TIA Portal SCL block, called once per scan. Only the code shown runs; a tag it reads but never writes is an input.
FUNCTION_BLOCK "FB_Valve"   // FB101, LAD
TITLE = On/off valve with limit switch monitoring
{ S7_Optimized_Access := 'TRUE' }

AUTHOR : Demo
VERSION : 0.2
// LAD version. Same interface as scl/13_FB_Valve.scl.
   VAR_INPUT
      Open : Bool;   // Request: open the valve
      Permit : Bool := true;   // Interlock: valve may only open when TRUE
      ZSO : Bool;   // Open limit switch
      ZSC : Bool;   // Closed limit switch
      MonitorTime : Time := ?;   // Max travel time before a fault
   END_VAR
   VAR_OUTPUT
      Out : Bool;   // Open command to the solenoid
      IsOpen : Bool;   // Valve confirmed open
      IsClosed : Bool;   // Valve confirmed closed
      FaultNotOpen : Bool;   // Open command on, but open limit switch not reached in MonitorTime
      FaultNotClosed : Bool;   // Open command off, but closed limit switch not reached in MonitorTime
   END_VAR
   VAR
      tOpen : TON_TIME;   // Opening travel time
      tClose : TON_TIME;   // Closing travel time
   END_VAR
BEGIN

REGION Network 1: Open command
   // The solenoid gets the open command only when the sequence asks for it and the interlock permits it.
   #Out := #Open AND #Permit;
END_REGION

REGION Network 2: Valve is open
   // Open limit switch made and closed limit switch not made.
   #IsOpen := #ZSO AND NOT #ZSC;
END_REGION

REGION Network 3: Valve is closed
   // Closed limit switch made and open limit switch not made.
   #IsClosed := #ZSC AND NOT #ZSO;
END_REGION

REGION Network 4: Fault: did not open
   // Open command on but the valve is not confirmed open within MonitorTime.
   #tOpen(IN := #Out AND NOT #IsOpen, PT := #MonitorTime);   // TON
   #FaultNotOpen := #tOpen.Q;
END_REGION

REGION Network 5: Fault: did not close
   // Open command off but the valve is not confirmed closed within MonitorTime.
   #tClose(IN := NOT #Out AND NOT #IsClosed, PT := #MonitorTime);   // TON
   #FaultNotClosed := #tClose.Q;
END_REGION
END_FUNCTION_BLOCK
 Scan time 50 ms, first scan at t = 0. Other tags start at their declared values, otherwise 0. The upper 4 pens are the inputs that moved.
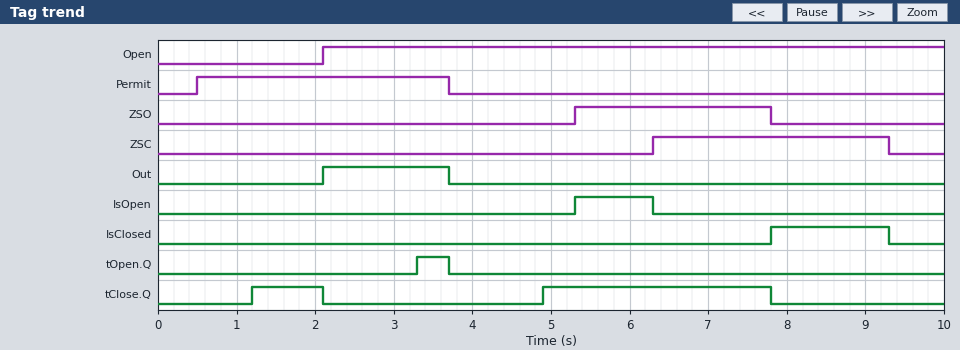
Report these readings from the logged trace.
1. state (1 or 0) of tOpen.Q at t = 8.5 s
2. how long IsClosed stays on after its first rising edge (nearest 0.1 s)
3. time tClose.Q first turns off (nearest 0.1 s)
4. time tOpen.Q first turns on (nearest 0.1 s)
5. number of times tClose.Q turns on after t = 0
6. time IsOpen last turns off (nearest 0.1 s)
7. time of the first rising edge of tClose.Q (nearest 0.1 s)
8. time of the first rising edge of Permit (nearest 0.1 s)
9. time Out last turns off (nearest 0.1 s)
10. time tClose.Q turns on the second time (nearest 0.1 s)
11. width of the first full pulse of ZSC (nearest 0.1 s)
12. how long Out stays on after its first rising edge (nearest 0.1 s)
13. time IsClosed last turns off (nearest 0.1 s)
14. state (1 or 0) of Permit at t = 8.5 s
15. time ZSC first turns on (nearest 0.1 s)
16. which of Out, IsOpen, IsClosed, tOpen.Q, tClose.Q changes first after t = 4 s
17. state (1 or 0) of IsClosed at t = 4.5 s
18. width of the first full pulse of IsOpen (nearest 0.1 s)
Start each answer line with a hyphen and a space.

- 0
- 1.5 s
- 2.1 s
- 3.3 s
- 2
- 6.3 s
- 1.2 s
- 0.5 s
- 3.7 s
- 4.9 s
- 3.0 s
- 1.6 s
- 9.3 s
- 0
- 6.3 s
- tClose.Q
- 0
- 1.0 s
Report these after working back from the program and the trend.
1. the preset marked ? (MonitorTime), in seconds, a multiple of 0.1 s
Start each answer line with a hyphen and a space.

- 1.2 s
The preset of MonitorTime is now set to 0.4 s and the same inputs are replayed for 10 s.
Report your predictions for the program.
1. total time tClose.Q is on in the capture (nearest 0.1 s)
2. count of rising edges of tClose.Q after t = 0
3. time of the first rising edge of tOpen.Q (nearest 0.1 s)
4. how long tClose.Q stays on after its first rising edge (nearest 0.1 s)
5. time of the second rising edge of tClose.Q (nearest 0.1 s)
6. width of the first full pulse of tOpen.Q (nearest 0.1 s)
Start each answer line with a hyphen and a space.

- 5.7 s
- 3
- 2.5 s
- 1.7 s
- 4.1 s
- 1.2 s
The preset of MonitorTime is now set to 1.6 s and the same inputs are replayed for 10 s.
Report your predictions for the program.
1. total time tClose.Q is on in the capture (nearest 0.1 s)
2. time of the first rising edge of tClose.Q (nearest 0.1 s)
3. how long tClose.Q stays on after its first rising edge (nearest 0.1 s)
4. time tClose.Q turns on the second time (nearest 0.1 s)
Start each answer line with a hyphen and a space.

- 3.0 s
- 1.6 s
- 0.5 s
- 5.3 s
